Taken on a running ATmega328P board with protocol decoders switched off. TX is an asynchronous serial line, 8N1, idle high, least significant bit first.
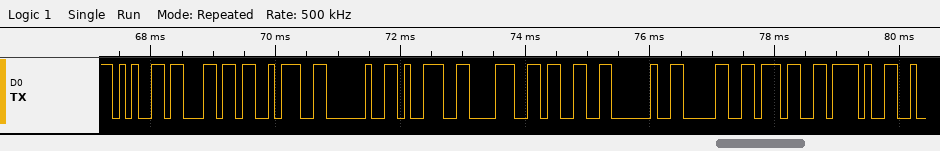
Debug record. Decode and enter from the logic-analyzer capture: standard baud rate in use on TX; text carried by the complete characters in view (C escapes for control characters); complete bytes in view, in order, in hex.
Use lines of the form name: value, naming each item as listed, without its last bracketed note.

standard baud rate in use on TX: 9600 baud
text carried by the complete characters in view: "el: 983 07/"
complete bytes in view, in order, in hex: 0x65 0x6C 0x3A 0x20 0x39 0x38 0x33 0x20 0x30 0x37 0x2F
